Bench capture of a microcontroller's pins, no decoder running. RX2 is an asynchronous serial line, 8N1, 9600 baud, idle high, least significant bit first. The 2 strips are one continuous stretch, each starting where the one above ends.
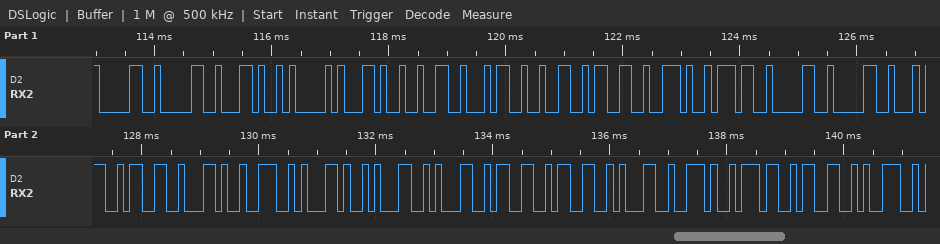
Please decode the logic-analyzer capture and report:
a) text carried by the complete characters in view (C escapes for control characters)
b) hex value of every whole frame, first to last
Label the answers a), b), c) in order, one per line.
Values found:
a) "00,A,2423.70043,N,11331.739"
b) 30 30 2C 41 2C 32 34 32 33 2E 37 30 30 34 33 2C 4E 2C 31 31 33 33 31 2E 37 33 39
